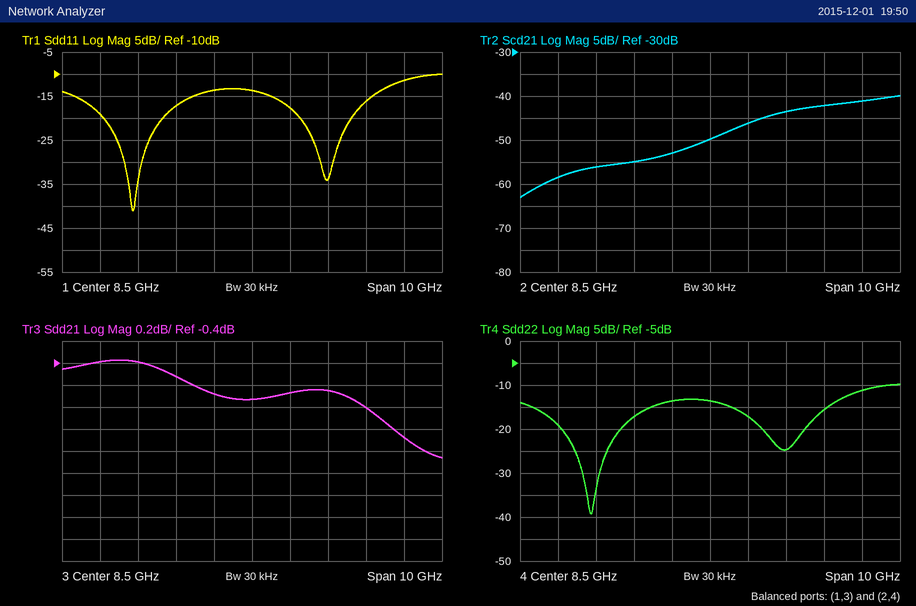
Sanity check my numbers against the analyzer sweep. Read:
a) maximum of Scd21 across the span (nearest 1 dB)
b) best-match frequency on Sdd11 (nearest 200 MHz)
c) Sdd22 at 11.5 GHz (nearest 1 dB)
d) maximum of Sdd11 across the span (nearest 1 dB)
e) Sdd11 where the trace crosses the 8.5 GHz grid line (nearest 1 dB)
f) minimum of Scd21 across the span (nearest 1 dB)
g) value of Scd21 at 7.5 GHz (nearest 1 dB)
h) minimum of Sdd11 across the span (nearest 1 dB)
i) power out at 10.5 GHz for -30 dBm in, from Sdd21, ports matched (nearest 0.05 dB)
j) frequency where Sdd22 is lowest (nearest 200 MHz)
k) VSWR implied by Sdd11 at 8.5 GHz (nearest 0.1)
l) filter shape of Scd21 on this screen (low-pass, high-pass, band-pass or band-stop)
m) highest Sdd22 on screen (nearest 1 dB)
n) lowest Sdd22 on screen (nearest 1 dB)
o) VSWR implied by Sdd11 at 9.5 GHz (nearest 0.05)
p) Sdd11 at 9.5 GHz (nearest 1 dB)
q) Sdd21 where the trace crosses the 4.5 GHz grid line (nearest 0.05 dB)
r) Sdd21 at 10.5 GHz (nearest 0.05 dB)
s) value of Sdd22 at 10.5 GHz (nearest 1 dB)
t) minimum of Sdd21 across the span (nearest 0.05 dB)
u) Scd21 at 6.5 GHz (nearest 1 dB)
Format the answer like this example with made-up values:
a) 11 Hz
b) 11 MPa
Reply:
a) -40 dB
b) 5.4 GHz
c) -16 dB
d) -10 dB
e) -14 dB
f) -63 dB
g) -53 dB
h) -41 dB
i) -30.65 dBm
j) 5.4 GHz
k) 1.5
l) high-pass
m) -10 dB
n) -39 dB
o) 1.30
p) -18 dB
q) -0.40 dB
r) -0.65 dB
s) -25 dB
t) -1.25 dB
u) -55 dB
